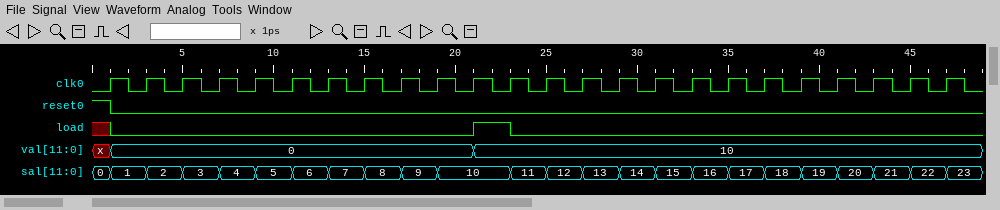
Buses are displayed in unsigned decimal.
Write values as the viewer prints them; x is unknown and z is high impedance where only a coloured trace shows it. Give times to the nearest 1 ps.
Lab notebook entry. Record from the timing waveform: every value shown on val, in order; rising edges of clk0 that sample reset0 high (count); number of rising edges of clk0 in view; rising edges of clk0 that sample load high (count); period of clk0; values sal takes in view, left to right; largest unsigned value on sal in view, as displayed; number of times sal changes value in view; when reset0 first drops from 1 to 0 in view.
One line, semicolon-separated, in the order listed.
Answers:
x, 0, 10; 1; 24; 1; 2 ps; 0, 1, 2, 3, 4, 5, 6, 7, 8, 9, 10, 11, 12, 13, 14, 15, 16, 17, 18, 19, 20, 21, 22, 23; 23; 23; 1 ps
